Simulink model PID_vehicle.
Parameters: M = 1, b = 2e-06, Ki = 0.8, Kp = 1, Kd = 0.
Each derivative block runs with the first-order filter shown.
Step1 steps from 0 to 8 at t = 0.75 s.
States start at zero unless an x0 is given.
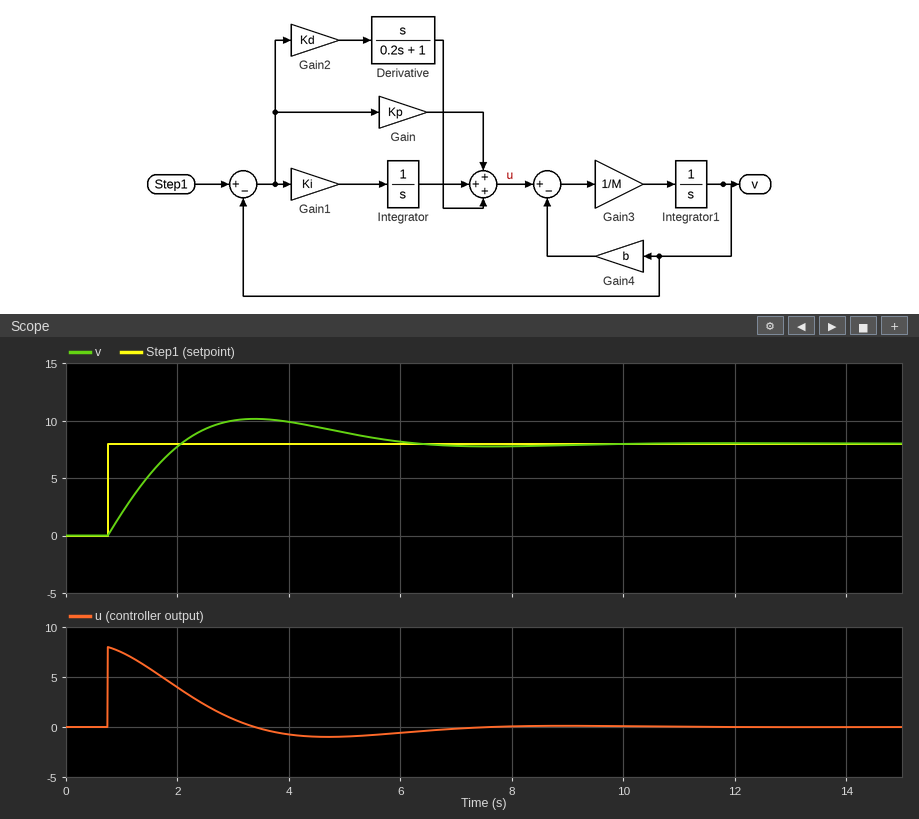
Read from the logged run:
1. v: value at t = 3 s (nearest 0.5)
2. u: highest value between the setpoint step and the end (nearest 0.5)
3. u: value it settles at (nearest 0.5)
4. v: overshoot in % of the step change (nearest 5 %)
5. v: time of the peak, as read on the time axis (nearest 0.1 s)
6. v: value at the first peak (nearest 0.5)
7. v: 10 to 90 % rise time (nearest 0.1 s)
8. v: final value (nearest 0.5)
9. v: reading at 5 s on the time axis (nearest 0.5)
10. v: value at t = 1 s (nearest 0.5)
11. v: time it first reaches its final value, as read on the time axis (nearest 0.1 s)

10.0
8.0
0.0
25 %
3.4 s
10.0
1.0 s
8.0
9.0
2.0
2.1 s
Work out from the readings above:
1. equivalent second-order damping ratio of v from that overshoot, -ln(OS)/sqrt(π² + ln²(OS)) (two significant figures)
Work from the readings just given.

0.40
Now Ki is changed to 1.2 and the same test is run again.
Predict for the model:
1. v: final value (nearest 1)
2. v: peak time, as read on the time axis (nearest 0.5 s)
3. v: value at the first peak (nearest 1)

8
3.0 s
11
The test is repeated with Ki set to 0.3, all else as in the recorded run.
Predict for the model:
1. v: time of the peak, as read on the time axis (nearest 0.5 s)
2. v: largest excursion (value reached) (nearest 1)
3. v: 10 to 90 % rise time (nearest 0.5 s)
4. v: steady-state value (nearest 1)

4.5 s
9
1.5 s
8
